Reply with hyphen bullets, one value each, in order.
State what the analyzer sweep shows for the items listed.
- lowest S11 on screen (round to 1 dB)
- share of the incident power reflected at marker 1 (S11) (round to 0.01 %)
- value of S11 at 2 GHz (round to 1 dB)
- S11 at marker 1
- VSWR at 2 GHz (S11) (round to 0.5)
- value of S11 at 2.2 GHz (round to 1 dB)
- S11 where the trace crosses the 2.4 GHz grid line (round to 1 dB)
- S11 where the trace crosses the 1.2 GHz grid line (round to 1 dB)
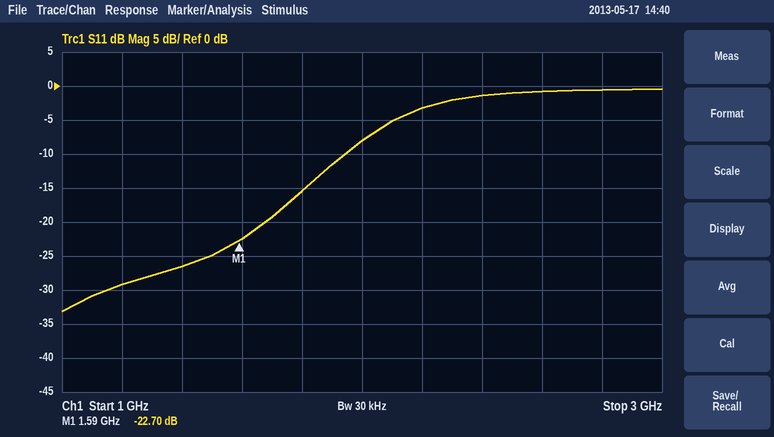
- -33 dB
- 0.54 %
- -8 dB
- -22.70 dB
- 2.5
- -3 dB
- -1 dB
- -29 dB
